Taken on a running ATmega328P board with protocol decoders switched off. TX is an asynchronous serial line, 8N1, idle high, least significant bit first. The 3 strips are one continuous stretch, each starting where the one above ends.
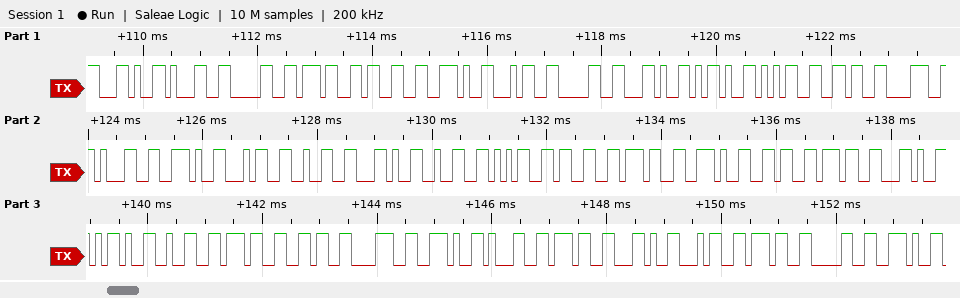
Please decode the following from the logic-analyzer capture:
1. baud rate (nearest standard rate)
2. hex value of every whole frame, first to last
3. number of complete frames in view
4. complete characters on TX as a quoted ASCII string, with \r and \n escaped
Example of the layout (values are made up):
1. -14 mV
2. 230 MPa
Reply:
1. 9600 baud
2. 2C 31 30 37 33 2E 34 30 2C 2D 35 36 38 31 2E 34 32 2C 32 35 33 37 2E 36 37 2C 2D 32 37 36 38 2E 31 37 2C 34 37 30 2E
3. 39
4. ",1073.40,-5681.42,2537.67,-2768.17,470."
